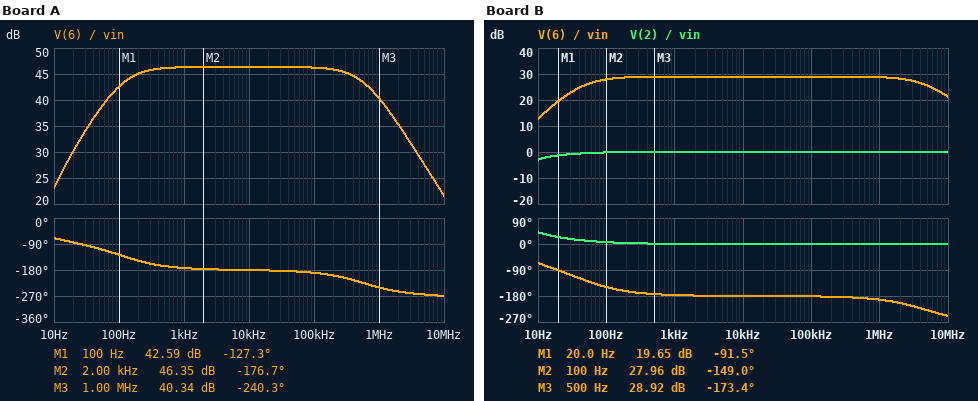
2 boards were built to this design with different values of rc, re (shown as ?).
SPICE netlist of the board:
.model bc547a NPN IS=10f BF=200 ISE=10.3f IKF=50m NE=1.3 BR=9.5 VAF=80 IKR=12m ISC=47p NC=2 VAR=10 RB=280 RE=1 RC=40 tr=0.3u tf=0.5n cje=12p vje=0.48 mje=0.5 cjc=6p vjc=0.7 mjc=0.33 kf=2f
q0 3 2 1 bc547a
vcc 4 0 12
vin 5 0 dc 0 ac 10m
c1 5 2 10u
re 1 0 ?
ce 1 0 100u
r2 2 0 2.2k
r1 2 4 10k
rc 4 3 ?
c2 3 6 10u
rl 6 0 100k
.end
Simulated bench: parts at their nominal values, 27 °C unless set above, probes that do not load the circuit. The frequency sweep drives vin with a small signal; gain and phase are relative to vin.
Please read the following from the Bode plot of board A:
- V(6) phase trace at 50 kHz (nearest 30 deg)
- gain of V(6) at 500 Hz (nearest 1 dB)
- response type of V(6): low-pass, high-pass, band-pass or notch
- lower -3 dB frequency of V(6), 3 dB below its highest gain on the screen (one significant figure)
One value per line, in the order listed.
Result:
-180 deg
46 dB
band-pass
100 Hz
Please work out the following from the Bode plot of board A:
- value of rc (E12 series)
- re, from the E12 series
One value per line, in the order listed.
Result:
3.3 kΩ
560 Ω
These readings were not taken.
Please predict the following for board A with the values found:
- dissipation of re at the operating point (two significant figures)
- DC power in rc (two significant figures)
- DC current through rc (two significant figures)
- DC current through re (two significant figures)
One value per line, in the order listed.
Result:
3.7 mW
21 mW
2.5 mA
2.6 mA
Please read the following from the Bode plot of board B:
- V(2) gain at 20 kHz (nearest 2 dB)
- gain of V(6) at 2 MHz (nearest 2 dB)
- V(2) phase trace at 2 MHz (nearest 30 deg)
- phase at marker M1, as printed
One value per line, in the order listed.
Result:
0 dB
28 dB
0 deg
-91.5 deg
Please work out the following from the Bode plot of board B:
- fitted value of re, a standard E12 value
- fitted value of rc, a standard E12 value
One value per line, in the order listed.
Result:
1.8 kΩ
1 kΩ
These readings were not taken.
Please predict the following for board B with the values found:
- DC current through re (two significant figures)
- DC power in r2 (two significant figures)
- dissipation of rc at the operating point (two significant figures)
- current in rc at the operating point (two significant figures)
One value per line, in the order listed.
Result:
830 µA
2.1 mW
680 µW
830 µA
